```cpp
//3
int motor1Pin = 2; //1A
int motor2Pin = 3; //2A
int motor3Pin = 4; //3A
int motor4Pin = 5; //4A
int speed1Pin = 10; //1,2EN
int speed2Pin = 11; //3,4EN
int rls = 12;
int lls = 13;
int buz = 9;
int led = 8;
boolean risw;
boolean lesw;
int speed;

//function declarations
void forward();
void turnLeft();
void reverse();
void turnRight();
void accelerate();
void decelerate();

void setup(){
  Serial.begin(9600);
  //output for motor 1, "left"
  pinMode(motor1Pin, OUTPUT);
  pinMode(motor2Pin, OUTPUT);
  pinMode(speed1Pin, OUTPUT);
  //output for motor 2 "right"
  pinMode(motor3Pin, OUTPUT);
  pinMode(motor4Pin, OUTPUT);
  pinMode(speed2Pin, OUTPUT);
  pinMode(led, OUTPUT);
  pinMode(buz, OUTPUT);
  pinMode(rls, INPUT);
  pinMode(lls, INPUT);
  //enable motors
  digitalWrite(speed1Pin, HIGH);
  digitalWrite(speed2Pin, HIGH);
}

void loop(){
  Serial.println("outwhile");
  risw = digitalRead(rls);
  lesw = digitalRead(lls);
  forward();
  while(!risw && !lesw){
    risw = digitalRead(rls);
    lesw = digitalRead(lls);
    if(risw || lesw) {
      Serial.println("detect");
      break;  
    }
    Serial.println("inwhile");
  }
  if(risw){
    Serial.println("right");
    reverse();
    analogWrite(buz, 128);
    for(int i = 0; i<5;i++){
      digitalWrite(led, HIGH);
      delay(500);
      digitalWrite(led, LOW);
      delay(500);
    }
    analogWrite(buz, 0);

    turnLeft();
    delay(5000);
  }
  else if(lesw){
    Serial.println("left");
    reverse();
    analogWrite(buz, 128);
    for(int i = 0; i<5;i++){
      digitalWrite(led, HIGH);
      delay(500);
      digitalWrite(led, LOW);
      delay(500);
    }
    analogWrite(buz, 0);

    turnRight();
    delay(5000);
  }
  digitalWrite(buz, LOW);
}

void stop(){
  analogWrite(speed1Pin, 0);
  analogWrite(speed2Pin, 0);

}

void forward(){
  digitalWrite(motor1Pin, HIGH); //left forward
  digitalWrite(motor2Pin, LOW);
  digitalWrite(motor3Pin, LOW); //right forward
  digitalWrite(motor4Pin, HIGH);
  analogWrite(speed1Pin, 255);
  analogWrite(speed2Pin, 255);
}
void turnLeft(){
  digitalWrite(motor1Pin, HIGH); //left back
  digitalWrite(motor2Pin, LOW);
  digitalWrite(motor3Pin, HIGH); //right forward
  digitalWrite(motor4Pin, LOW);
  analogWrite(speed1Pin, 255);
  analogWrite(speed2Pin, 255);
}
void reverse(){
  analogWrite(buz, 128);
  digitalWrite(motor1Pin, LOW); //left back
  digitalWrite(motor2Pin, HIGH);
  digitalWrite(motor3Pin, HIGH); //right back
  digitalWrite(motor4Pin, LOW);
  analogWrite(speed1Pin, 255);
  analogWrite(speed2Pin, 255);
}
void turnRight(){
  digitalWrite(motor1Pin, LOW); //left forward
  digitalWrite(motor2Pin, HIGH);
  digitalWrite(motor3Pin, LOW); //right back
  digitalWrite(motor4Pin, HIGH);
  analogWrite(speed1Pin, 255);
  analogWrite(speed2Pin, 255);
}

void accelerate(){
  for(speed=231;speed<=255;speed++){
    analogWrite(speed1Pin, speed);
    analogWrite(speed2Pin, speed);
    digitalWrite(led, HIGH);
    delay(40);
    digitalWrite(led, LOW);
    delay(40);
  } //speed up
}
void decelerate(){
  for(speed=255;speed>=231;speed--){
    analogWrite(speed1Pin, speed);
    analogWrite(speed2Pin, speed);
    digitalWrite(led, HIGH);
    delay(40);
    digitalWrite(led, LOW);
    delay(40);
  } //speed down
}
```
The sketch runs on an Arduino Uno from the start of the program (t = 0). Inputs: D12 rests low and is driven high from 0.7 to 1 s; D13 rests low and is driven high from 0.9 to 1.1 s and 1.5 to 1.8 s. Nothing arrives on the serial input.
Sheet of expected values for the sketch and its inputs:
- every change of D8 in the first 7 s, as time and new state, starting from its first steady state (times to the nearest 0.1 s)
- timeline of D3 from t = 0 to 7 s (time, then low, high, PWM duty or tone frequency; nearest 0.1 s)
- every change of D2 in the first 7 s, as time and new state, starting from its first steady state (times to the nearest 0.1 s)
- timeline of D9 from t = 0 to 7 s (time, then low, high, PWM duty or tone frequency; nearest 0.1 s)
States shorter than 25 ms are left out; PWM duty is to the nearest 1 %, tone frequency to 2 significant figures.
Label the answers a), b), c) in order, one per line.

a) 0 s low; 0.7 s high; 1.2 s low; 1.7 s high; 2.2 s low; 2.7 s high; 3.2 s low; 3.7 s high; 4.2 s low; 4.7 s high; 5.2 s low
b) 0 s low; 0.7 s high; 5.7 s low
c) 0 s high; 0.7 s low; 5.7 s high
d) 0 s low; 0.7 s PWM 50 %; 5.7 s low
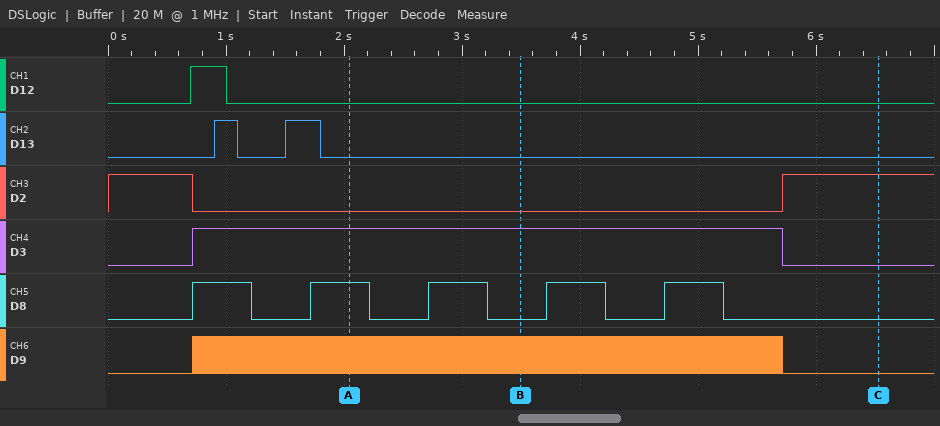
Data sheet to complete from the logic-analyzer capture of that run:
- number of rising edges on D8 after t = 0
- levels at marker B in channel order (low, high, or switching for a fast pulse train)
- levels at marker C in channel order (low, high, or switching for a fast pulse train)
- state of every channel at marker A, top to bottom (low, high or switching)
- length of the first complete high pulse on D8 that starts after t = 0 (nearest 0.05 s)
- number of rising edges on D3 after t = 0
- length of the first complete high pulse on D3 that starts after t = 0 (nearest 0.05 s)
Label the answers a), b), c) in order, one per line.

a) 5
b) D12 low, D13 low, D2 low, D3 high, D8 low, D9 switching
c) D12 low, D13 low, D2 high, D3 low, D8 low, D9 low
d) D12 low, D13 low, D2 low, D3 high, D8 high, D9 switching
e) 0.50 s
f) 1
g) 5.00 s
